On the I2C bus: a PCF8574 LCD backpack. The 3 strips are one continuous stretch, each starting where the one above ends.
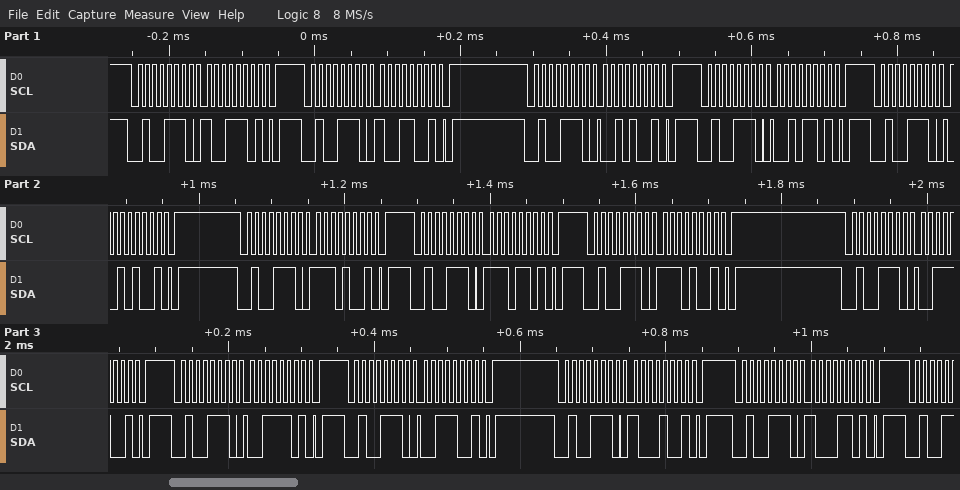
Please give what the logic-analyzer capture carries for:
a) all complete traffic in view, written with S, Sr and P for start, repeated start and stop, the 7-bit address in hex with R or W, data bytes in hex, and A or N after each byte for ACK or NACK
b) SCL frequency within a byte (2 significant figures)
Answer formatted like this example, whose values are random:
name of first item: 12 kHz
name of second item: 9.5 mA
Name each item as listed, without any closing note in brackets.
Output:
all complete traffic in view, written with S, Sr and P for start, repeated start and stop, the 7-bit address in hex with R or W, data bytes in hex, and A or N after each byte for ACK or NACK: S 27W A 9D A P S 27W A 99 A P S 27W A 29 A P S 27W A 2D A P S 27W A 29 A P S 27W A E9 A P S 27W A ED A P S 27W A E9 A P S 27W A 39 A P S 27W A 3D A P S 27W A 39 A P S 27W A 89 A P S 27W A 8D A P
SCL frequency within a byte: 100 kHz
